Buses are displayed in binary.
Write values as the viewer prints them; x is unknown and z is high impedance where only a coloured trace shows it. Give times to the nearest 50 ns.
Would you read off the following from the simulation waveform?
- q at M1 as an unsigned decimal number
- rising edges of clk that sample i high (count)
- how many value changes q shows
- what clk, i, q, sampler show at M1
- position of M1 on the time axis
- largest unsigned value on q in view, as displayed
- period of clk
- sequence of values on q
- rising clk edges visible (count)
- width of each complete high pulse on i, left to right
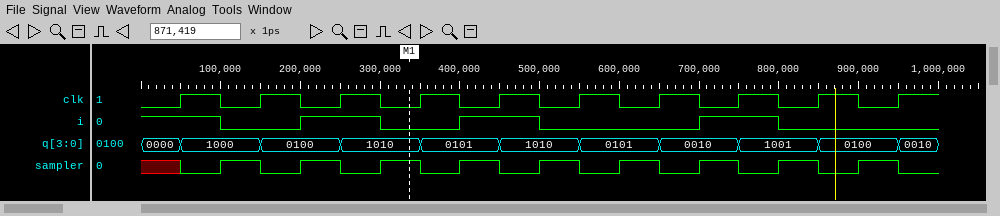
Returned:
10
4
10
clk=0, i=0, q=1010, sampler=1
350 ns
1010
100 ns
0000, 1000, 0100, 1010, 0101, 1010, 0101, 0010, 1001, 0100, 0010
10
100 ns, 100 ns, 100 ns
